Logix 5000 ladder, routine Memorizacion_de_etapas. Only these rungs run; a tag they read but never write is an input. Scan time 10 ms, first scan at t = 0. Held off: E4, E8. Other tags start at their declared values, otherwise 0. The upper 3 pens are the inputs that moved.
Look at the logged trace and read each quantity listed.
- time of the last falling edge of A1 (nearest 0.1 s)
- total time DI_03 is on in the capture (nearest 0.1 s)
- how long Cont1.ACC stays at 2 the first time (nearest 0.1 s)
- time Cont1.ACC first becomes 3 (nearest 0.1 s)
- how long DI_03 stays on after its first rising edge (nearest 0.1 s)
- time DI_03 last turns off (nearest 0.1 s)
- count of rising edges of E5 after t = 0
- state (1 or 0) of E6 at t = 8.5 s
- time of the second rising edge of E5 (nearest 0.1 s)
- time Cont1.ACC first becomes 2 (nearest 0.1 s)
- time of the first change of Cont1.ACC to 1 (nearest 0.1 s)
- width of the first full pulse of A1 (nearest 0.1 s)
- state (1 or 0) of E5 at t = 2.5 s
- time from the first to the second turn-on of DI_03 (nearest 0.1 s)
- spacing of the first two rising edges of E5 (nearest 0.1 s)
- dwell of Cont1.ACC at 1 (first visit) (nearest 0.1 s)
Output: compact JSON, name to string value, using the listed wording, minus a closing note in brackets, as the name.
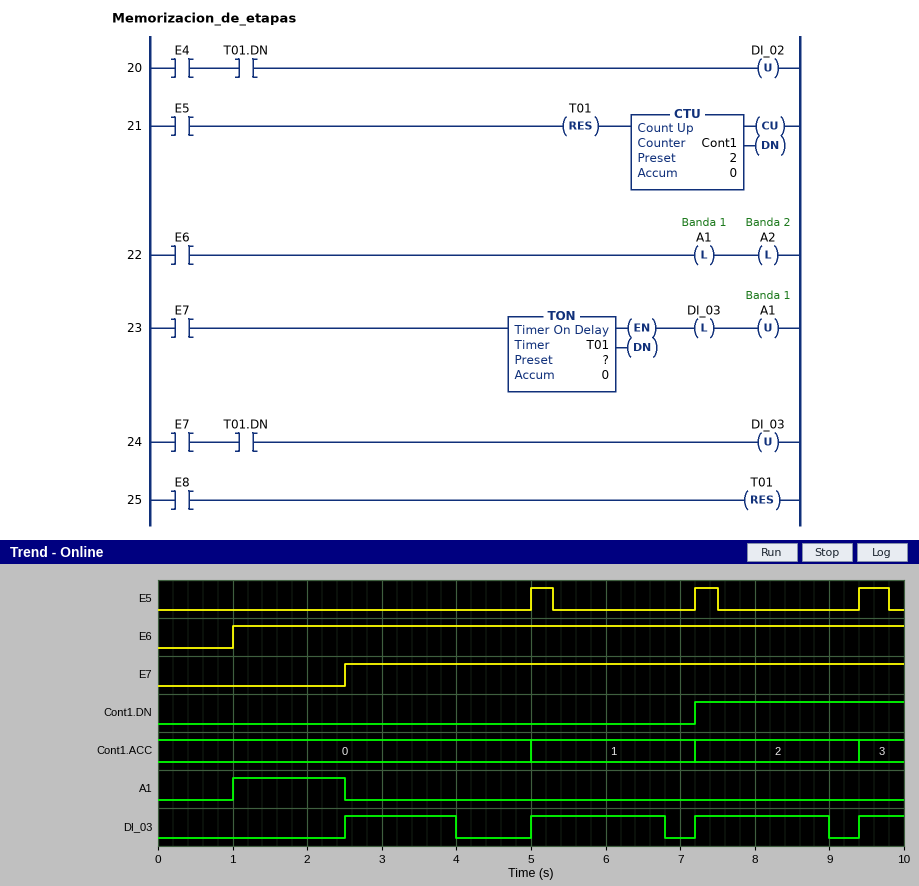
{"time of the last falling edge of A1": "2.5 s", "total time DI_03 is on in the capture": "5.7 s", "how long Cont1.ACC stays at 2 the first time": "2.2 s", "time Cont1.ACC first becomes 3": "9.4 s", "how long DI_03 stays on after its first rising edge": "1.5 s", "time DI_03 last turns off": "9.0 s", "count of rising edges of E5 after t = 0": "3", "state (1 or 0) of E6 at t = 8.5 s": "1", "time of the second rising edge of E5": "7.2 s", "time Cont1.ACC first becomes 2": "7.2 s", "time of the first change of Cont1.ACC to 1": "5.0 s", "width of the first full pulse of A1": "1.5 s", "state (1 or 0) of E5 at t = 2.5 s": "0", "time from the first to the second turn-on of DI_03": "2.5 s", "spacing of the first two rising edges of E5": "2.2 s", "dwell of Cont1.ACC at 1 (first visit)": "2.2 s"}
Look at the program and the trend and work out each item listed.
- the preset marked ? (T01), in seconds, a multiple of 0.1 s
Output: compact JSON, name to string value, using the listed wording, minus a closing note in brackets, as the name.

{"the preset marked ? (T01), in seconds, a multiple of 0.1 s": "1.5 s"}
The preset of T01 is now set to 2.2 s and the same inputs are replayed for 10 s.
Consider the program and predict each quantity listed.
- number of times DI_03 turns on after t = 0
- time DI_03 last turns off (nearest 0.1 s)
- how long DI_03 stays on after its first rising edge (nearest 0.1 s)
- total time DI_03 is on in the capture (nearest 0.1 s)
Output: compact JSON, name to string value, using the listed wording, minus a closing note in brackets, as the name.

{"number of times DI_03 turns on after t = 0": "2", "time DI_03 last turns off": "4.7 s", "how long DI_03 stays on after its first rising edge": "2.2 s", "total time DI_03 is on in the capture": "7.2 s"}
